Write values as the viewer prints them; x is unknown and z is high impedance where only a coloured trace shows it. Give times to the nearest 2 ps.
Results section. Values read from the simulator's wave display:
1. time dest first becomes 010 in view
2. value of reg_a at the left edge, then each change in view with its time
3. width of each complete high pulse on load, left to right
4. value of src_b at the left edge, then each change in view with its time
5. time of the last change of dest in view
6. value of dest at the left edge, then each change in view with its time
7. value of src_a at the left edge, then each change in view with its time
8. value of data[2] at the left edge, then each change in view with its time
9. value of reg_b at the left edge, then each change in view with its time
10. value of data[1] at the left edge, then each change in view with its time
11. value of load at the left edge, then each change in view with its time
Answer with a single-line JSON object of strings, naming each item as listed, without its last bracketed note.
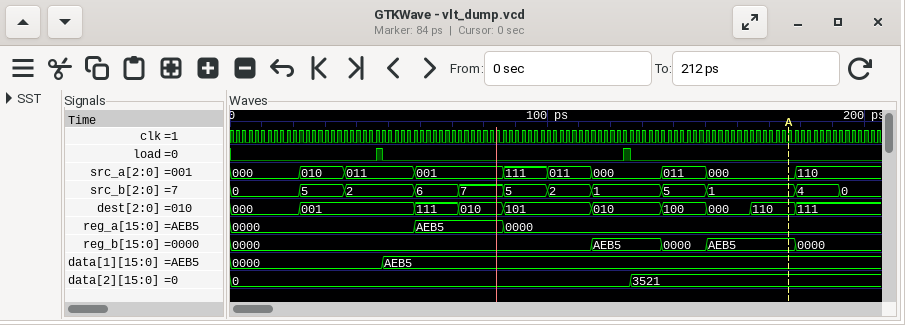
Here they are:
{"time dest first becomes 010 in view": "72 ps", "value of reg_a at the left edge, then each change in view with its time": "0000, AEB5 at 58 ps, 0000 at 86 ps", "width of each complete high pulse on load, left to right": "2 ps, 2 ps", "value of src_b at the left edge, then each change in view with its time": "0, 5 at 22 ps, 2 at 36 ps, 6 at 58 ps, 7 at 72 ps, 5 at 86 ps, 2 at 100 ps, 1 at 114 ps, 5 at 136 ps, 1 at 150 ps, 4 at 178 ps, 0 at 192 ps", "time of the last change of dest in view": "178 ps", "value of dest at the left edge, then each change in view with its time": "000, 001 at 22 ps, 111 at 58 ps, 010 at 72 ps, 101 at 86 ps, 010 at 114 ps, 100 at 136 ps, 000 at 150 ps, 110 at 164 ps, 111 at 178 ps", "value of src_a at the left edge, then each change in view with its time": "000, 010 at 22 ps, 011 at 36 ps, 001 at 58 ps, 111 at 86 ps, 011 at 100 ps, 000 at 114 ps, 011 at 136 ps, 000 at 150 ps, 110 at 178 ps", "value of data[2] at the left edge, then each change in view with its time": "0, 3521 at 126 ps", "value of reg_b at the left edge, then each change in view with its time": "0000, AEB5 at 114 ps, 0000 at 136 ps, AEB5 at 150 ps, 0000 at 178 ps", "value of data[1] at the left edge, then each change in view with its time": "0000, AEB5 at 48 ps", "value of load at the left edge, then each change in view with its time": "0, 1 at 46 ps, 0 at 48 ps, 1 at 124 ps, 0 at 126 ps"}
